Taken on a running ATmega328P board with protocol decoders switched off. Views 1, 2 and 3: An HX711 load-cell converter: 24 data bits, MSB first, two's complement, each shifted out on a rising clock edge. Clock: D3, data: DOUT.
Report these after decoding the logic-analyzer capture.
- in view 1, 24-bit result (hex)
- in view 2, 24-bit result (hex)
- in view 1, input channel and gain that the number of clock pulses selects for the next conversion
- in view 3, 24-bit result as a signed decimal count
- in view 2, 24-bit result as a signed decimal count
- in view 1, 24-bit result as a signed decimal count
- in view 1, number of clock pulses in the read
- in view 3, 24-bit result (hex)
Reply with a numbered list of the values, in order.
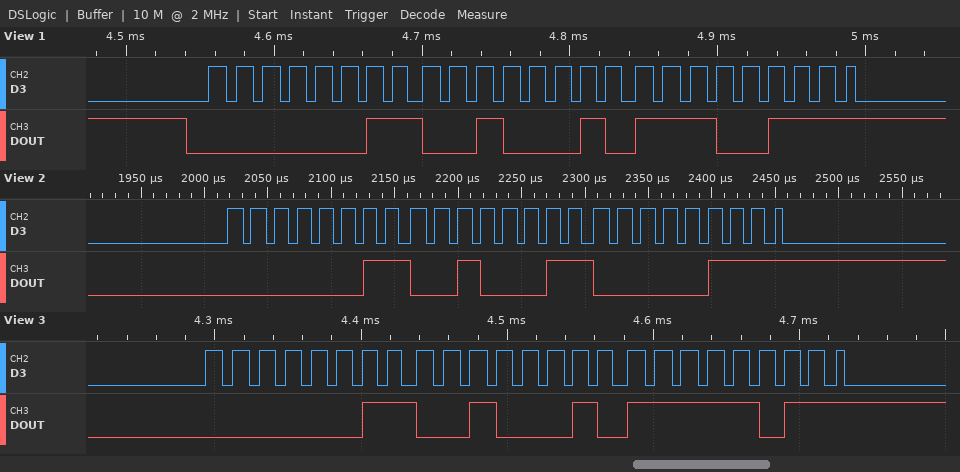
1. 0x0322E7
2. 0x032307
3. channel A, gain 128
4. 205563
5. 205575
6. 205543
7. 25
8. 0x0322FB
